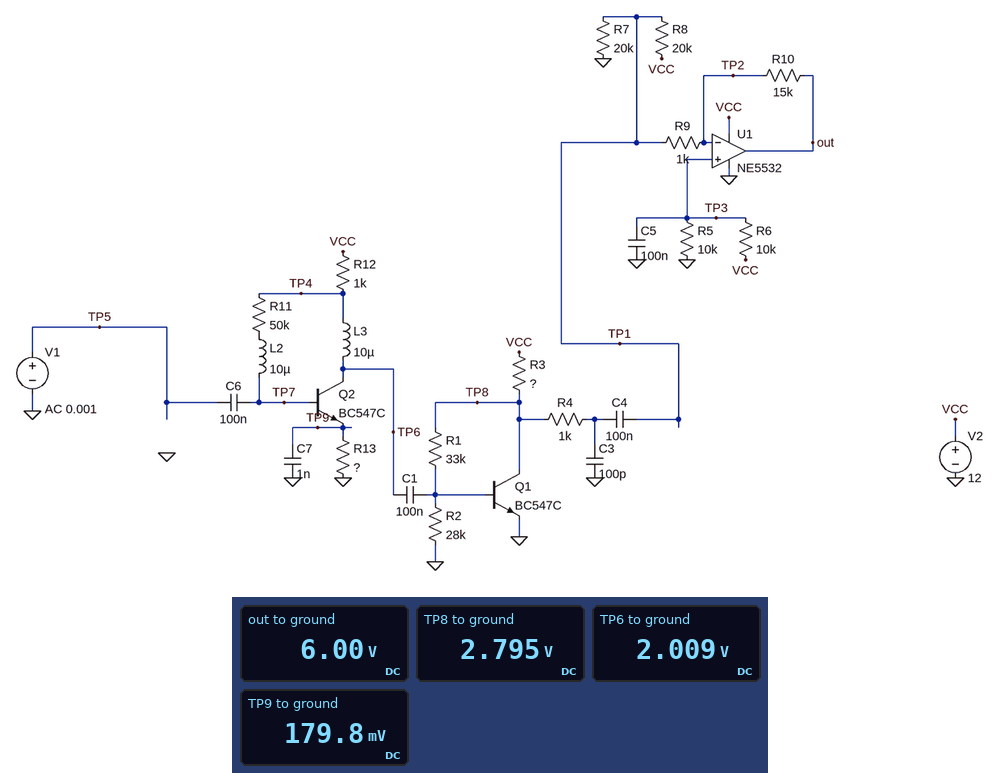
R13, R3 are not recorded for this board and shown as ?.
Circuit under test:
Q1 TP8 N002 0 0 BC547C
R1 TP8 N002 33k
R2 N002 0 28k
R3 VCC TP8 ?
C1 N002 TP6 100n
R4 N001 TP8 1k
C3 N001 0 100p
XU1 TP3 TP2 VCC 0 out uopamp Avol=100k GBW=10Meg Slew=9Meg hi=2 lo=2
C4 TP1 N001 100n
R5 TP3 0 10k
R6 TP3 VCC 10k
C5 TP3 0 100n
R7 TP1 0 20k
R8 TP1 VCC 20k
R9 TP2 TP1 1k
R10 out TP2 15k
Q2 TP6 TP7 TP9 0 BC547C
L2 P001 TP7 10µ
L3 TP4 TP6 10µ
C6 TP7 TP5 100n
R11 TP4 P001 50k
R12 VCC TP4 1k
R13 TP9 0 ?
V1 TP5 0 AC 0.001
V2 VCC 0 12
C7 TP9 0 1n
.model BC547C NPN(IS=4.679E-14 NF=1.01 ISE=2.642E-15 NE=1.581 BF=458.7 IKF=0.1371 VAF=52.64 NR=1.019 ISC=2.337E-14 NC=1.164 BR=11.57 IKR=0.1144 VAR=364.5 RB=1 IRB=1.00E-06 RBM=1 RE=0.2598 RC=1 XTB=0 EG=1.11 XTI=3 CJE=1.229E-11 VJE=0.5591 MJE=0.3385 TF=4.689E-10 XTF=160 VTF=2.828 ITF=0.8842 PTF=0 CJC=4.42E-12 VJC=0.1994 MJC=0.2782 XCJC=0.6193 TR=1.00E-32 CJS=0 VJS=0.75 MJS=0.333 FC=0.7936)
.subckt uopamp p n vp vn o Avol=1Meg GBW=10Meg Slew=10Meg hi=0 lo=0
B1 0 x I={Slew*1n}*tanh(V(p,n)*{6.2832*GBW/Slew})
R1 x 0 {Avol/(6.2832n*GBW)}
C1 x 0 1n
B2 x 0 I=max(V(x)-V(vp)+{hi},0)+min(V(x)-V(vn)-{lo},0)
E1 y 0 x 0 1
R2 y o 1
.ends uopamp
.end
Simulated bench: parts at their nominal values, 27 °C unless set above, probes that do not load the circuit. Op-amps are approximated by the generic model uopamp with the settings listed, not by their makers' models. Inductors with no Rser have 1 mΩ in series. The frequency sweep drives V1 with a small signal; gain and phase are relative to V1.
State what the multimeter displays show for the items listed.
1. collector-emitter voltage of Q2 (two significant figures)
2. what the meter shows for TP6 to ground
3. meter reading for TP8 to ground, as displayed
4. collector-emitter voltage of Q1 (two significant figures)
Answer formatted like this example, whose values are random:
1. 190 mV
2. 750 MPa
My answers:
1. 1.8 V
2. 2.009 V
3. 2.795 V
4. 2.8 V
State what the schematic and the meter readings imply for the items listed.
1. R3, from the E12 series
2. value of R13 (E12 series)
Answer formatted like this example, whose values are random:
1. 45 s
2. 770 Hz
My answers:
1. 560 Ω
2. 18 Ω
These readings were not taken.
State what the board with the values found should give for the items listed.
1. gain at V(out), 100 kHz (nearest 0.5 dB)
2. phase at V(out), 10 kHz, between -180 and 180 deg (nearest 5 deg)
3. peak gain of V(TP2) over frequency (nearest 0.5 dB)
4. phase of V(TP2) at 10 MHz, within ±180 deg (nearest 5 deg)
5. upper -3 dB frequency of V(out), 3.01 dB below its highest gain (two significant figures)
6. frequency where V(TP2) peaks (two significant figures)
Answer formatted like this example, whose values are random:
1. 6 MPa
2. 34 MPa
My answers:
1. 78.0 dB
2. -165 deg
3. 55.0 dB
4. -120 deg
5. 970 kHz
6. 1.2 MHz
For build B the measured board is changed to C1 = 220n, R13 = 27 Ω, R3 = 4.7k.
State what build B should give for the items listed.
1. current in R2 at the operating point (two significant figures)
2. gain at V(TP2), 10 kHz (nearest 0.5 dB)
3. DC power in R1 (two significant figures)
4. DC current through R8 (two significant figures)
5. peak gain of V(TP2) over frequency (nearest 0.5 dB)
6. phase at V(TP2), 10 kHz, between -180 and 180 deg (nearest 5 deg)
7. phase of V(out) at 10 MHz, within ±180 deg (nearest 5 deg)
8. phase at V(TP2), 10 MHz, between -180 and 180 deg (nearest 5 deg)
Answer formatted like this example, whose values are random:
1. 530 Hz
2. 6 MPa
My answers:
1. 23 µA
2. 15.0 dB
3. 25 µW
4. 300 µA
5. 52.5 dB
6. 100 deg
7. -20 deg
8. -110 deg
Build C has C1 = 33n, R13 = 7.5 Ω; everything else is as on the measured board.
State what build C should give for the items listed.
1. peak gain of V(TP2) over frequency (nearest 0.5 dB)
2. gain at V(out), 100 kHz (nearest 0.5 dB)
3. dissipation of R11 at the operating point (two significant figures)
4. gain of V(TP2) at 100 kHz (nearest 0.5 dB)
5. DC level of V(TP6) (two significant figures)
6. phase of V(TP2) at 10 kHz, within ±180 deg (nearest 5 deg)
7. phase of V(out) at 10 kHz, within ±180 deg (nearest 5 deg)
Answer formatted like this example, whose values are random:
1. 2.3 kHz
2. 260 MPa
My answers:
1. 61.0 dB
2. 84.0 dB
3. 27 µW
4. 44.0 dB
5. 1.9 V
6. 125 deg
7. -145 deg
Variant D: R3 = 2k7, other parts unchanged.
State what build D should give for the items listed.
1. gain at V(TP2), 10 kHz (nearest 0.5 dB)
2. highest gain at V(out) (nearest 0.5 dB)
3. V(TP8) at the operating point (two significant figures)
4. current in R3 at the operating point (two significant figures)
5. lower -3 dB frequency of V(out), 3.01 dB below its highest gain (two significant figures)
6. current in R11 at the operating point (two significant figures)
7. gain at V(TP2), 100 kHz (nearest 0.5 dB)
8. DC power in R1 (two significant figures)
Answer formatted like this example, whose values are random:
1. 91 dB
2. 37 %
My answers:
1. 18.5 dB
2. 78.5 dB
3. 1.7 V
4. 3.8 mA
5. 1.4 kHz
6. 23 µA
7. 38.5 dB
8. 33 µW
